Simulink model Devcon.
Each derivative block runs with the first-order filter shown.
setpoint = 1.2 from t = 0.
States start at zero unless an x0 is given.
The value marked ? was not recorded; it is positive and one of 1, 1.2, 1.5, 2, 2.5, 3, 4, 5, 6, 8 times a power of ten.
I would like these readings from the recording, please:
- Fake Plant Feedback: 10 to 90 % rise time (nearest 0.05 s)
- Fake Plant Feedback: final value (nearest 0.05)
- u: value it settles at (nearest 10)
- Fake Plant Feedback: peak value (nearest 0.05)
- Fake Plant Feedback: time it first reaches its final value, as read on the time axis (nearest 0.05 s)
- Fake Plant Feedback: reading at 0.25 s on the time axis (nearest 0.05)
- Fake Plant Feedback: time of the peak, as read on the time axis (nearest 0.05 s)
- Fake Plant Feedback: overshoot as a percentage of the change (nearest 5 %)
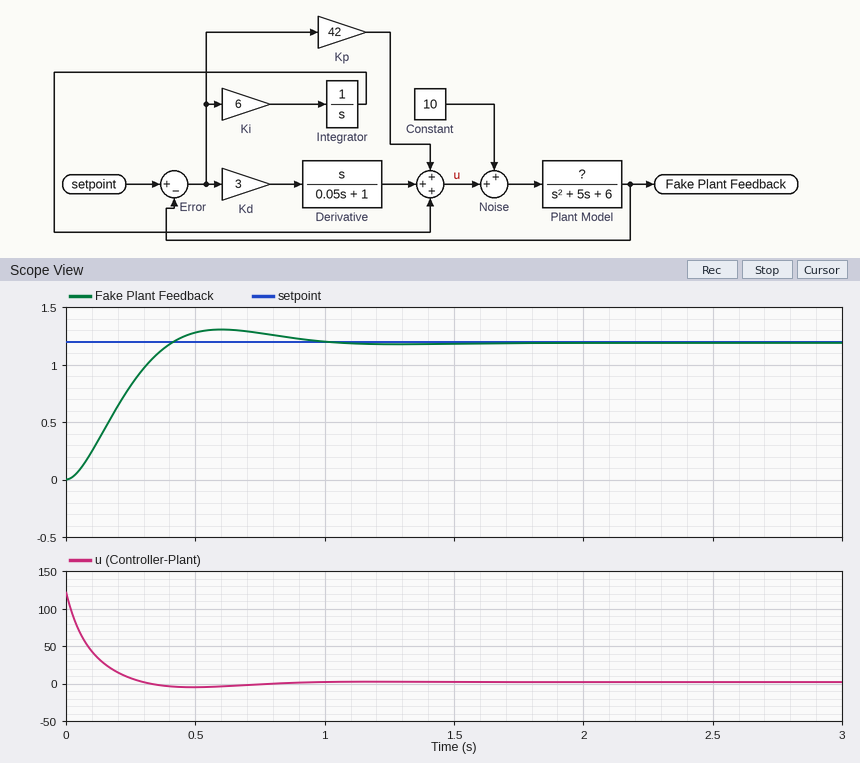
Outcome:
0.30 s
1.20
0
1.30
0.40 s
0.80
0.60 s
10 %
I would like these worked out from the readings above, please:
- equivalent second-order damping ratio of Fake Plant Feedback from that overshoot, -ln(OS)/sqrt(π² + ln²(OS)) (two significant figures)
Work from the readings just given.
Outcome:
0.59
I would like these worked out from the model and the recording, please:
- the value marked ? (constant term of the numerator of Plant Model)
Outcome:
0.6
